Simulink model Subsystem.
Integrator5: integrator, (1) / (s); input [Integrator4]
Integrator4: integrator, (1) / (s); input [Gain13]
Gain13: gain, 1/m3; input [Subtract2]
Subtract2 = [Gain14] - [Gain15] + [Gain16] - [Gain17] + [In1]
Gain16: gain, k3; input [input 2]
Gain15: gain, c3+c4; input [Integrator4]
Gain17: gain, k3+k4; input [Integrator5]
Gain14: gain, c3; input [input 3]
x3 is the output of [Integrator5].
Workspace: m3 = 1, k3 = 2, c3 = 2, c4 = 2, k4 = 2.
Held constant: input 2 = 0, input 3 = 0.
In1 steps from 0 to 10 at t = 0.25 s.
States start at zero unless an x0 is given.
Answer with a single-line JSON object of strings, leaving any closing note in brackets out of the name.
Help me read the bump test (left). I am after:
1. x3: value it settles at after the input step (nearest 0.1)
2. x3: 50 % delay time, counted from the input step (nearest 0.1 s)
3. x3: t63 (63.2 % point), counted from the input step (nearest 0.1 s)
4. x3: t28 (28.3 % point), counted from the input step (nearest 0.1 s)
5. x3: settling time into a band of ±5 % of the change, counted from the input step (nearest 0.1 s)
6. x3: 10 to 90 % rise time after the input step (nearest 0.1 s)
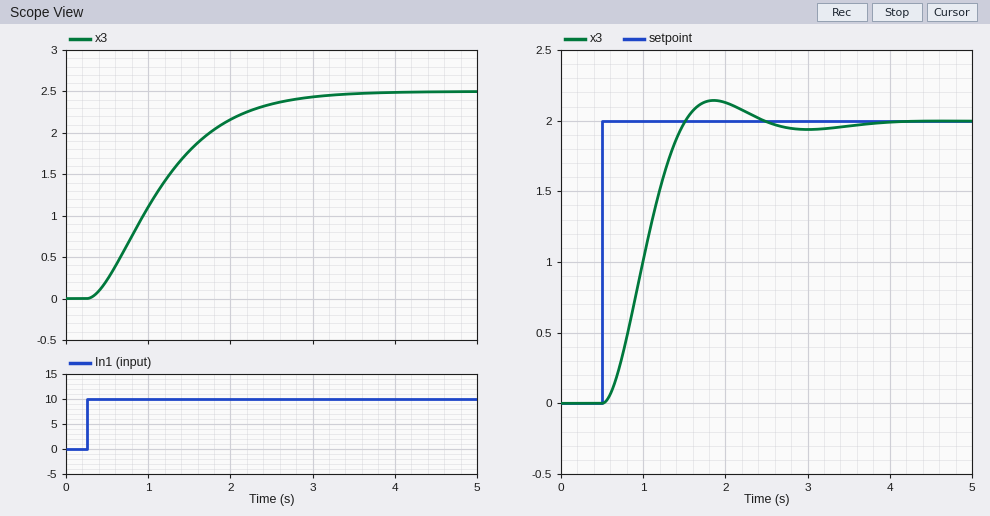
{"x3: value it settles at after the input step": "2.5", "x3: 50 % delay time, counted from the input step": "0.8 s", "x3: t63 (63.2 % point), counted from the input step": "1.1 s", "x3: t28 (28.3 % point), counted from the input step": "0.5 s", "x3: settling time into a band of ±5 % of the change, counted from the input step": "2.4 s", "x3: 10 to 90 % rise time after the input step": "1.7 s"}
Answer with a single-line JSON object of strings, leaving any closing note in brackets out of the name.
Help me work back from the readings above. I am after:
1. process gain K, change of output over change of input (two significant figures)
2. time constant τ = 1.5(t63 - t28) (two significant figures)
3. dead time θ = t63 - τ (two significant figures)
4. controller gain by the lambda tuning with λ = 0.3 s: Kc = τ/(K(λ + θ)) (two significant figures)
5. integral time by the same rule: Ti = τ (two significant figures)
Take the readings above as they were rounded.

{"process gain K, change of output over change of input": "0.25", "time constant τ = 1.5(t63 - t28)": "0.90 s", "dead time θ = t63 - τ": "0.20 s", "controller gain by the lambda tuning with λ = 0.3 s: Kc = τ/(K(λ + θ))": "7.2", "integral time by the same rule: Ti = τ": "0.90 s"}
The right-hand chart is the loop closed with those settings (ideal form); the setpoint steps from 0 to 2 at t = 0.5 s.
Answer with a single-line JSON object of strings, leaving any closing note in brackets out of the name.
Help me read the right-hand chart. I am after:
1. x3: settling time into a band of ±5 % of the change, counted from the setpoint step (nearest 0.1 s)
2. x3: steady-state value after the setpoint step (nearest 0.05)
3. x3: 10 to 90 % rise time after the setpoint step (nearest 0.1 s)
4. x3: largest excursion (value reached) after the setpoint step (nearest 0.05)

{"x3: settling time into a band of ±5 % of the change, counted from the setpoint step": "1.6 s", "x3: steady-state value after the setpoint step": "2.00", "x3: 10 to 90 % rise time after the setpoint step": "0.7 s", "x3: largest excursion (value reached) after the setpoint step": "2.15"}
